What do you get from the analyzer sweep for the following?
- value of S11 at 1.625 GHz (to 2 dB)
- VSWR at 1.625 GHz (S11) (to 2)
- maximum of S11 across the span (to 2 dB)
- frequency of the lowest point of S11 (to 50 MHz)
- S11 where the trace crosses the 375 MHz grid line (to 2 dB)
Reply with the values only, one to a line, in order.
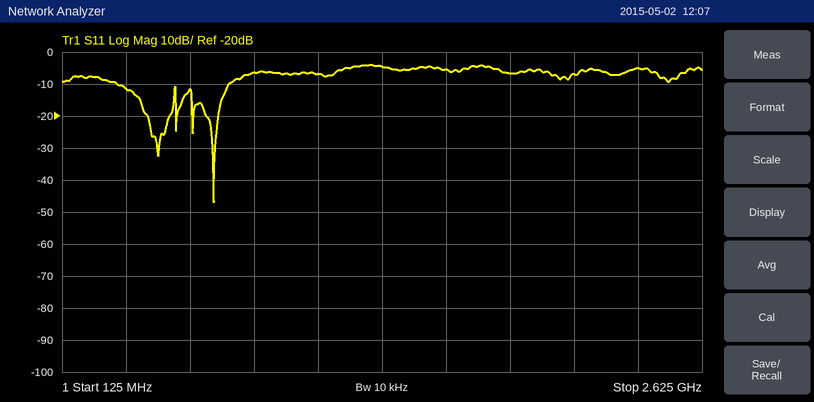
-6 dB
4
-4 dB
700 MHz
-12 dB
